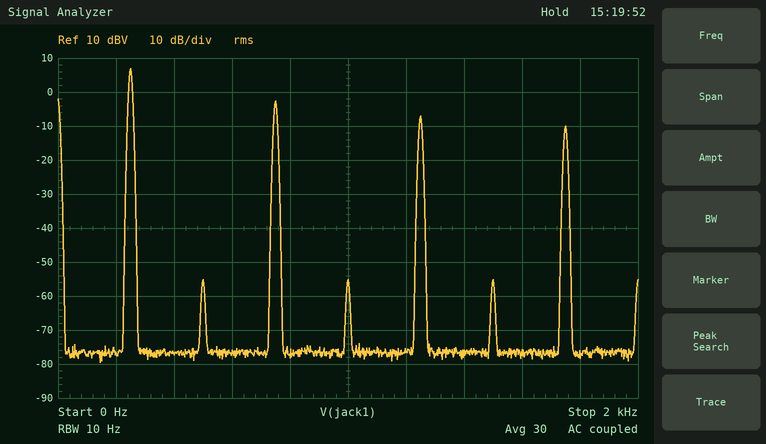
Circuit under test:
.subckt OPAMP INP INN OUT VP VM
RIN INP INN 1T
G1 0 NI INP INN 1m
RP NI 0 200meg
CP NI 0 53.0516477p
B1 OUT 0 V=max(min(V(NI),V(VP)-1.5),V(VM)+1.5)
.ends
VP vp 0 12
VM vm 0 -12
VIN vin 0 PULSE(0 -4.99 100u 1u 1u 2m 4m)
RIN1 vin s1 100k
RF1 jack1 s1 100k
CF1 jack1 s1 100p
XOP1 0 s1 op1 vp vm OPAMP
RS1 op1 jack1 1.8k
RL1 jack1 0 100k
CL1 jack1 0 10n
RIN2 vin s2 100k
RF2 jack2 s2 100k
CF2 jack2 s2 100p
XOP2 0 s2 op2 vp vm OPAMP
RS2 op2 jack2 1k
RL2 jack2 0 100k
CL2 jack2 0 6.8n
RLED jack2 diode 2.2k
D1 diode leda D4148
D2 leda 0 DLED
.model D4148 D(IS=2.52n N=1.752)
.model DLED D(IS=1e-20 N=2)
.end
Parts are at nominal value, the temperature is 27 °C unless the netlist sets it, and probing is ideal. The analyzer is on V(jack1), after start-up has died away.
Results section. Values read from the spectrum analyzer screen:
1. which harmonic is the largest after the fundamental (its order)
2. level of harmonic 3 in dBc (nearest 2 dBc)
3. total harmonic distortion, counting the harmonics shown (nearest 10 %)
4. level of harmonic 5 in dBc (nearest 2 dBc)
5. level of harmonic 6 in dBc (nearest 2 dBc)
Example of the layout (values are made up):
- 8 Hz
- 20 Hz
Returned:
- 3
- -10 dBc
- 40 %
- -14 dBc
- -62 dBc
